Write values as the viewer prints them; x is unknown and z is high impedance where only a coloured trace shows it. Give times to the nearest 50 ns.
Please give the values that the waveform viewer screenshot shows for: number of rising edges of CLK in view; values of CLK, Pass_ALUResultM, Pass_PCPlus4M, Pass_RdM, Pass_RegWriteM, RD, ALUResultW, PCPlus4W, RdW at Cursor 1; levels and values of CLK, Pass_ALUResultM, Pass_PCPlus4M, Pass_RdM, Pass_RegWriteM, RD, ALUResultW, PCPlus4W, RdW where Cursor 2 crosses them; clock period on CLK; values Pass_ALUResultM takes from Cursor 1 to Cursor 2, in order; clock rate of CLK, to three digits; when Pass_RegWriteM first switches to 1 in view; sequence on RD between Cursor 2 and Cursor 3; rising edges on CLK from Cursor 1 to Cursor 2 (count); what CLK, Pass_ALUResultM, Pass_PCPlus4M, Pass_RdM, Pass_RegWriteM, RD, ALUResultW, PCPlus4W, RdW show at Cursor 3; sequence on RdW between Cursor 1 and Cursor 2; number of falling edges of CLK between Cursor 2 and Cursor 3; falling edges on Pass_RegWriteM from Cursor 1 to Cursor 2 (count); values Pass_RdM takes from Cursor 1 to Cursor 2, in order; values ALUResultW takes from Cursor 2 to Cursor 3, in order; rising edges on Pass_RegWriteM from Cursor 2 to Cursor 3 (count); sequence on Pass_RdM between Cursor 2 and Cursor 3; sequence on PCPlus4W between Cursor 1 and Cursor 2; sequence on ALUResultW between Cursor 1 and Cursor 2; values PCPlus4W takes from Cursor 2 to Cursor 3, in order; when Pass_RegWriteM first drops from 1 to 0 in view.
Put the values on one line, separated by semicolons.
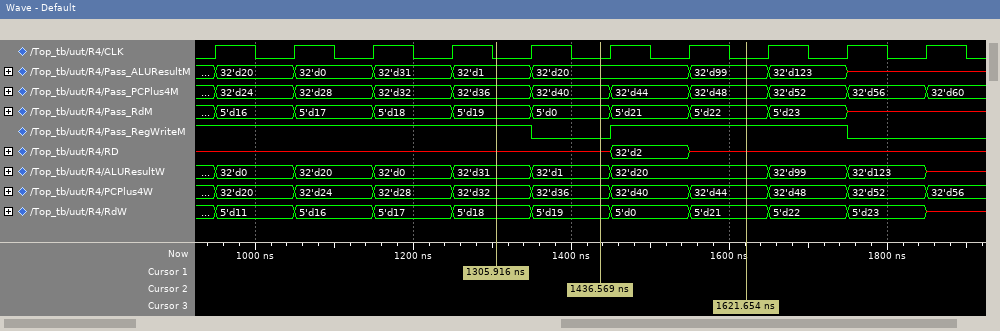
10; CLK=0, Pass_ALUResultM=32'd1, Pass_PCPlus4M=32'd36, Pass_RdM=5'd19, Pass_RegWriteM=1, RD=x, ALUResultW=32'd31, PCPlus4W=32'd32, RdW=5'd18; CLK=0, Pass_ALUResultM=32'd20, Pass_PCPlus4M=32'd40, Pass_RdM=5'd0, Pass_RegWriteM=0, RD=x, ALUResultW=32'd1, PCPlus4W=32'd36, RdW=5'd19; 100 ns; 32'd1, 32'd20; 10.0 MHz; 1450 ns; x, 32'd2, x; 1; CLK=0, Pass_ALUResultM=32'd99, Pass_PCPlus4M=32'd48, Pass_RdM=5'd22, Pass_RegWriteM=1, RD=x, ALUResultW=32'd20, PCPlus4W=32'd44, RdW=5'd21; 5'd18, 5'd19; 2; 1; 5'd19, 5'd0; 32'd1, 32'd20; 1; 5'd0, 5'd21, 5'd22; 32'd32, 32'd36; 32'd31, 32'd1; 32'd36, 32'd40, 32'd44; 1350 ns
